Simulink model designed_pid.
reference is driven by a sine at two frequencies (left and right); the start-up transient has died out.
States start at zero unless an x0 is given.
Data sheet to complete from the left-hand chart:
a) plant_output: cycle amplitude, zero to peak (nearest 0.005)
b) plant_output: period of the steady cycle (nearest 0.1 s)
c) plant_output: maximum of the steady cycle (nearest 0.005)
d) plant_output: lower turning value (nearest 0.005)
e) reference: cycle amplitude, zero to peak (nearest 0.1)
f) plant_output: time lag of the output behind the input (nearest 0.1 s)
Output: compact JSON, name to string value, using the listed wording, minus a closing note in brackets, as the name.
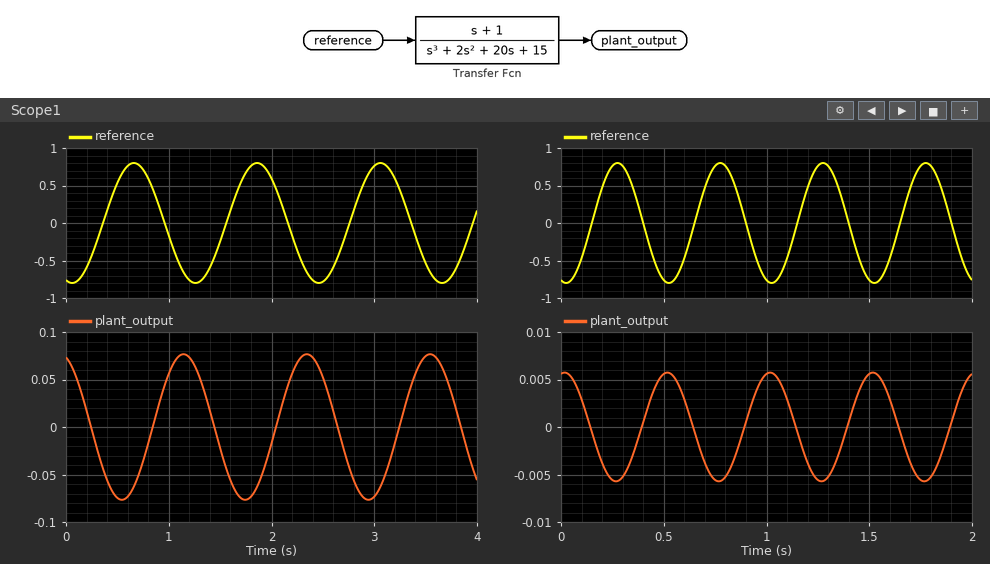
{"plant_output: cycle amplitude, zero to peak": "0.075", "plant_output: period of the steady cycle": "1.2 s", "plant_output: maximum of the steady cycle": "0.075", "plant_output: lower turning value": "-0.075", "reference: cycle amplitude, zero to peak": "0.8", "plant_output: time lag of the output behind the input": "0.5 s"}
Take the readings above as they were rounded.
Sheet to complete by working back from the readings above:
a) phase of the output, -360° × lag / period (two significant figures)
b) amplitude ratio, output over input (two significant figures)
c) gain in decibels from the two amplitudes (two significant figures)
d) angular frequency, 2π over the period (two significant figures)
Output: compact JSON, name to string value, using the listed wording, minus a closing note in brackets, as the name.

{"phase of the output, -360° × lag / period": "-150°", "amplitude ratio, output over input": "0.094", "gain in decibels from the two amplitudes": "-21 dB", "angular frequency, 2π over the period": "5.2 rad/s"}
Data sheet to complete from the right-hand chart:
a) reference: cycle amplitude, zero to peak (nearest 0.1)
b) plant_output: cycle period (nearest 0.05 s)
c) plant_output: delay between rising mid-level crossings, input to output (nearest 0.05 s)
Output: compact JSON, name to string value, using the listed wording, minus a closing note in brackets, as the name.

{"reference: cycle amplitude, zero to peak": "0.8", "plant_output: cycle period": "0.50 s", "plant_output: delay between rising mid-level crossings, input to output": "0.25 s"}
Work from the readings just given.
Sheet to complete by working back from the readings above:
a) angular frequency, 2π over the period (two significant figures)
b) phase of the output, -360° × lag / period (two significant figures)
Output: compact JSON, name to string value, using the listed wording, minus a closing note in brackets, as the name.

{"angular frequency, 2π over the period": "13 rad/s", "phase of the output, -360° × lag / period": "-180°"}
